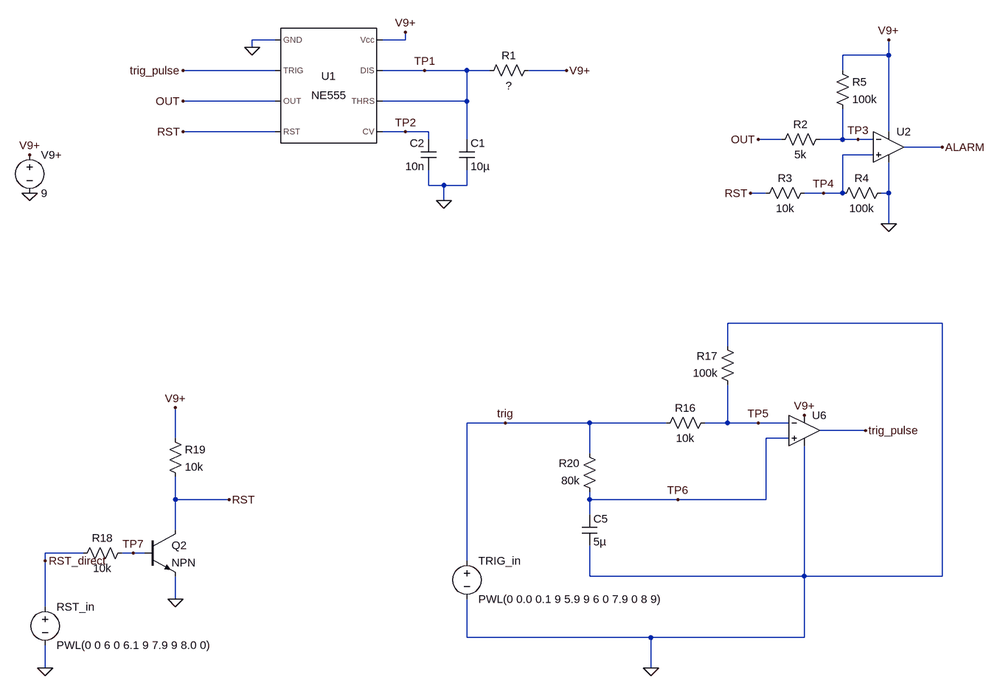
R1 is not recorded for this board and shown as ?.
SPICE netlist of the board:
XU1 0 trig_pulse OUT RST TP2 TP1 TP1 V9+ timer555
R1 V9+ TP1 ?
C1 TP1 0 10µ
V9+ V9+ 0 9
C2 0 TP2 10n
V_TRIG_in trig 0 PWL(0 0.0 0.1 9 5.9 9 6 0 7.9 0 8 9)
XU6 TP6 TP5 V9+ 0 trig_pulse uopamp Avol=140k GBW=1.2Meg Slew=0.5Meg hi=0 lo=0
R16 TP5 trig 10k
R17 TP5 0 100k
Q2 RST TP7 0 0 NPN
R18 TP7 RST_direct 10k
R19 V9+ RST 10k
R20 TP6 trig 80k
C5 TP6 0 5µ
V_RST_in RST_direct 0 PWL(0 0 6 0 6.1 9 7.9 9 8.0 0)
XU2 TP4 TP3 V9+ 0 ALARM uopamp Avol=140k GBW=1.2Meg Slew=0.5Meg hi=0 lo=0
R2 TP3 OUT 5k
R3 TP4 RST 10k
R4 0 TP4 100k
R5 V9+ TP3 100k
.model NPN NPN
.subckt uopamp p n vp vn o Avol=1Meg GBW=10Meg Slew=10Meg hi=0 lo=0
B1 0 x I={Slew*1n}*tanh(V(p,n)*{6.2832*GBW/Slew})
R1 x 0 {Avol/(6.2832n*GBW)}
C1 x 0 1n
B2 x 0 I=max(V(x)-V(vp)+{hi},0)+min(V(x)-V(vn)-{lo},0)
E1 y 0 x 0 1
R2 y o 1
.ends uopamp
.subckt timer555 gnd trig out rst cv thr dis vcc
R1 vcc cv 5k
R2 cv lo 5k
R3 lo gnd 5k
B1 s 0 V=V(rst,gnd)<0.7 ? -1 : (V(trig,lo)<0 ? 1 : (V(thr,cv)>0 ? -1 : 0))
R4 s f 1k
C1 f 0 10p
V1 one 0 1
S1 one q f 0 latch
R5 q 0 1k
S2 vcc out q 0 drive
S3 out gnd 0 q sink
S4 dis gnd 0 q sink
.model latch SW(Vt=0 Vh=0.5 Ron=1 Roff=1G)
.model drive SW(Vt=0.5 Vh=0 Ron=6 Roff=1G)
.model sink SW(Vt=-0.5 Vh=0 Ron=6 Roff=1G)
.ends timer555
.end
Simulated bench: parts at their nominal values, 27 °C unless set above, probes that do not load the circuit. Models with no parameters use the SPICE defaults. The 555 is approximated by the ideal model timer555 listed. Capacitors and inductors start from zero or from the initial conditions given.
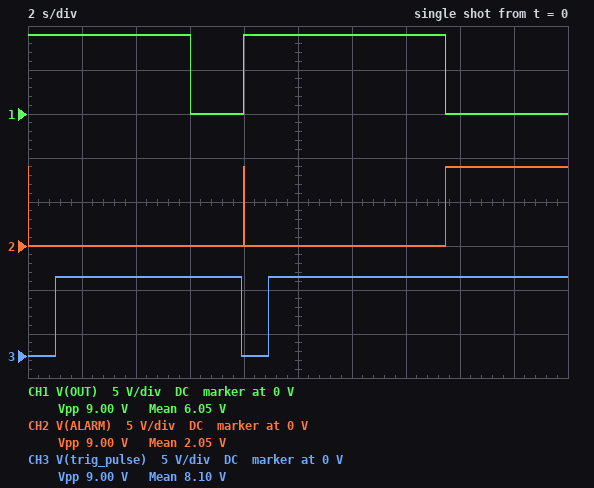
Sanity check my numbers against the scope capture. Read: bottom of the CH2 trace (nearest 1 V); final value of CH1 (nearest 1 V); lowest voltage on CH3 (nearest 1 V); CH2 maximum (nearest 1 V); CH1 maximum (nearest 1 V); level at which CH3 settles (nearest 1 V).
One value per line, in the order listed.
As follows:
0 V
0 V
0 V
9 V
9 V
9 V
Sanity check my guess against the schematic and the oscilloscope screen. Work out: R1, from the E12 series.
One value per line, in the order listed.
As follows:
680 kΩ
